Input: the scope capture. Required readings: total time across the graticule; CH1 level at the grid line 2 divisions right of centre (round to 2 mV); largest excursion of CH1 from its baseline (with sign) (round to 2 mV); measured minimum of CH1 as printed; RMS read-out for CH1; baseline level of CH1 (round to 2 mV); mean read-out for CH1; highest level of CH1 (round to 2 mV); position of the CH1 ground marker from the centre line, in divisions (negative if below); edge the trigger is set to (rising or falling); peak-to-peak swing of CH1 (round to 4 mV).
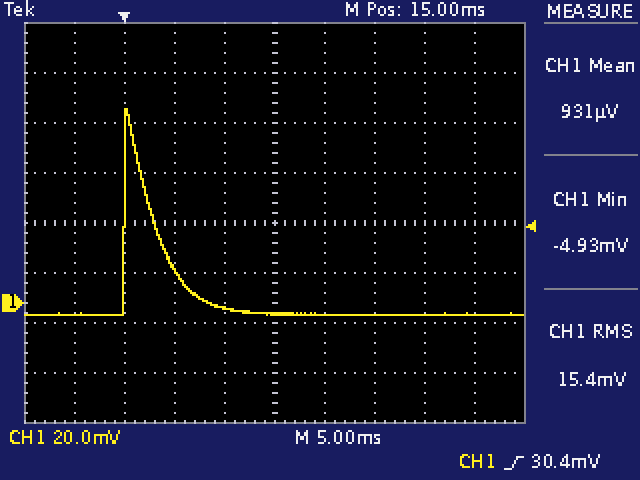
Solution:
50 ms
-4 mV
+82 mV
-4.93 mV
15.4 mV
-4 mV
931 µV
78 mV
-1.6 div
rising
84 mV
